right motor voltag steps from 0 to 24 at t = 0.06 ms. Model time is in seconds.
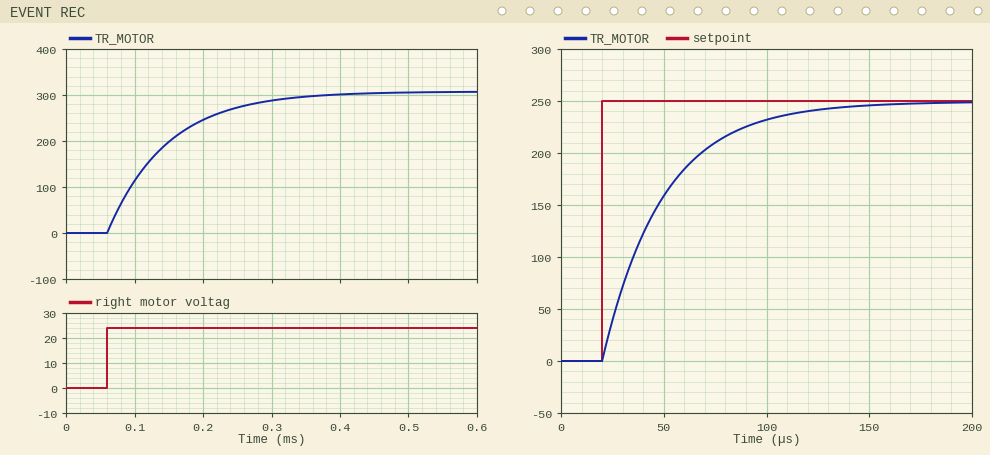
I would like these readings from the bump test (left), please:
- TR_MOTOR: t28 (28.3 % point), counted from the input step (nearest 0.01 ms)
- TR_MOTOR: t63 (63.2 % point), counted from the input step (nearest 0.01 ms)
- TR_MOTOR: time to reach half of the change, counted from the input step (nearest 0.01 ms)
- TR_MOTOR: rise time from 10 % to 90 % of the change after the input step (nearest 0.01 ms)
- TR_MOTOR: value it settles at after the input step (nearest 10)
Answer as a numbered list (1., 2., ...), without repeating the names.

1. 0.03 ms
2. 0.09 ms
3. 0.06 ms
4. 0.19 ms
5. 310
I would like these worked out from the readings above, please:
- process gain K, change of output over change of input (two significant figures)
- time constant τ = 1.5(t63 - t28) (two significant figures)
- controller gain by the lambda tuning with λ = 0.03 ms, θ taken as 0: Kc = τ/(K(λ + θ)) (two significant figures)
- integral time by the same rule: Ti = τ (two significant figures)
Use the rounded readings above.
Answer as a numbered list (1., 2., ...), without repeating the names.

1. 13
2. 0.090 ms
3. 0.23
4. 0.090 ms
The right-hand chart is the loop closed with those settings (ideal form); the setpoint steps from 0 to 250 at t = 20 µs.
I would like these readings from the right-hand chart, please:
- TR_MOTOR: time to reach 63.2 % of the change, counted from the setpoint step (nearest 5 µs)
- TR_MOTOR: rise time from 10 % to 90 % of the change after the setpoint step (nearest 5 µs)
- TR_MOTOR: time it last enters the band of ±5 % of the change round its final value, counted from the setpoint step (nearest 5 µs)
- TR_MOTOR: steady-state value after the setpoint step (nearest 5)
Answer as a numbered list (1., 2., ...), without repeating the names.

1. 30 µs
2. 65 µs
3. 90 µs
4. 250
